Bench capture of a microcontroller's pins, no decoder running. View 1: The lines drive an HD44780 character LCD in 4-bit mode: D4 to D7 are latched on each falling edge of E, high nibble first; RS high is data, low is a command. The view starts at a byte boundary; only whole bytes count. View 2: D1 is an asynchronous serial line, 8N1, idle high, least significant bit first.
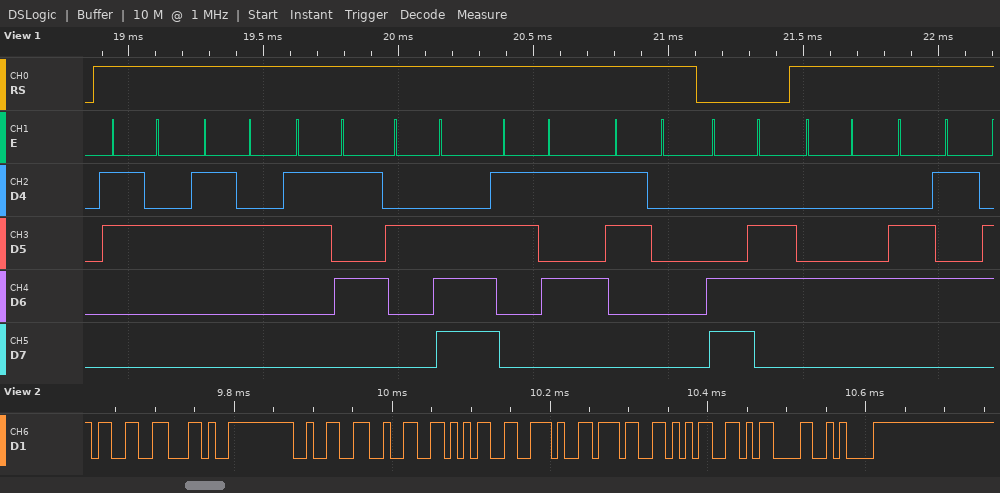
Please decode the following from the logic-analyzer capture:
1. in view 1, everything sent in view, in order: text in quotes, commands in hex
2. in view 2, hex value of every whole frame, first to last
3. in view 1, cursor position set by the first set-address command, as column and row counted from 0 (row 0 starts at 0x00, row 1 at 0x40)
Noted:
"225.50" 0xC6 "De"
33 2C 32 32 35 2E 37 35 0D 0A
column 6, row 1
